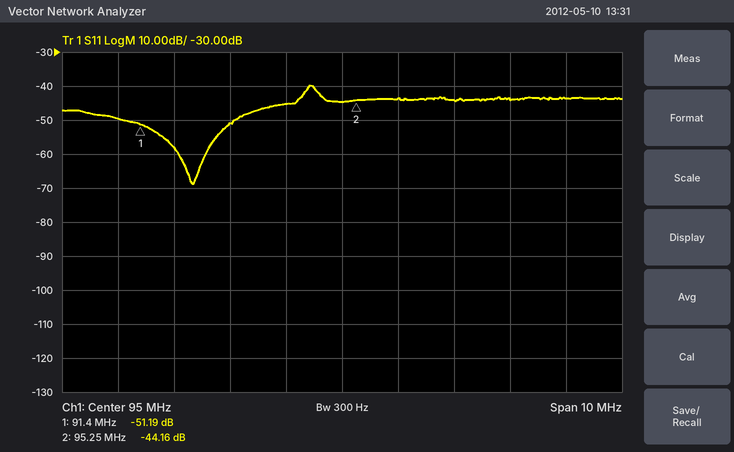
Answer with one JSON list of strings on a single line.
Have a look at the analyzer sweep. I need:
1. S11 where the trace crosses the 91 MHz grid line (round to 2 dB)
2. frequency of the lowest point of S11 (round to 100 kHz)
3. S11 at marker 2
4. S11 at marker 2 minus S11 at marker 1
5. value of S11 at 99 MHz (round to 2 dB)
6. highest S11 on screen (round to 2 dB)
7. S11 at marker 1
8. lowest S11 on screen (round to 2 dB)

["-50 dB", "92.3 MHz", "-44.16 dB", "7.03 dB", "-44 dB", "-40 dB", "-51.19 dB", "-68 dB"]
